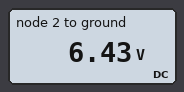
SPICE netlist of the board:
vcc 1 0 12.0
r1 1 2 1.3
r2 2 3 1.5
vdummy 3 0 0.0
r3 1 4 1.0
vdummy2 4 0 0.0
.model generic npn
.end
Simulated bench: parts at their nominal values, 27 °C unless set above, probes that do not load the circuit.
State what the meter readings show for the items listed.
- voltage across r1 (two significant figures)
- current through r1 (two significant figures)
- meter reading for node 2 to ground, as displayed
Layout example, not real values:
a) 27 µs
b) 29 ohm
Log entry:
a) 5.6 V
b) 4.3 A
c) 6.43 V
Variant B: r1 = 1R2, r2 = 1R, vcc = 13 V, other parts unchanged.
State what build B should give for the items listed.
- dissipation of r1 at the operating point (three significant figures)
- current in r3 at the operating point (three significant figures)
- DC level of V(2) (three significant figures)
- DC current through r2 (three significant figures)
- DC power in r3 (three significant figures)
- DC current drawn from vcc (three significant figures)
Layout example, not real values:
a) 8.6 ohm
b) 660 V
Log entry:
a) 41.9 W
b) 13.0 A
c) 5.91 V
d) 5.91 A
e) 169 W
f) 18.9 A
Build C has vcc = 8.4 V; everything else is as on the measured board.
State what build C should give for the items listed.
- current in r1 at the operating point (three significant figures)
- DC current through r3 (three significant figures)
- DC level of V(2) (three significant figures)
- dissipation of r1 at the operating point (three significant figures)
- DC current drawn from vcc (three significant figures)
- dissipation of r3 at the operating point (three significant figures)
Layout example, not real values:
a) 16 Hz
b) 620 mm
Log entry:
a) 3.00 A
b) 8.40 A
c) 4.50 V
d) 11.7 W
e) 11.4 A
f) 70.6 W
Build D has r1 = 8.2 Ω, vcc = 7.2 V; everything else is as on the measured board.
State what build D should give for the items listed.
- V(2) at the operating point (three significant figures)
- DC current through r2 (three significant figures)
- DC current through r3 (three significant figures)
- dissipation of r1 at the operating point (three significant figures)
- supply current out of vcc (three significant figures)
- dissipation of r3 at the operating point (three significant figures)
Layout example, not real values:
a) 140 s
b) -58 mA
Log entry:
a) 1.11 V
b) 742 mA
c) 7.20 A
d) 4.52 W
e) 7.94 A
f) 51.8 W
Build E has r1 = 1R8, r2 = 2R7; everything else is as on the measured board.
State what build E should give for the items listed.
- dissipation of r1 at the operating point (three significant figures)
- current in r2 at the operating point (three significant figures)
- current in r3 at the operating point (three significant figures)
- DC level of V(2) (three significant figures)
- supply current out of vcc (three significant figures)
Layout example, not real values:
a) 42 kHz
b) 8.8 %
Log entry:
a) 12.8 W
b) 2.67 A
c) 12.0 A
d) 7.20 V
e) 14.7 A
